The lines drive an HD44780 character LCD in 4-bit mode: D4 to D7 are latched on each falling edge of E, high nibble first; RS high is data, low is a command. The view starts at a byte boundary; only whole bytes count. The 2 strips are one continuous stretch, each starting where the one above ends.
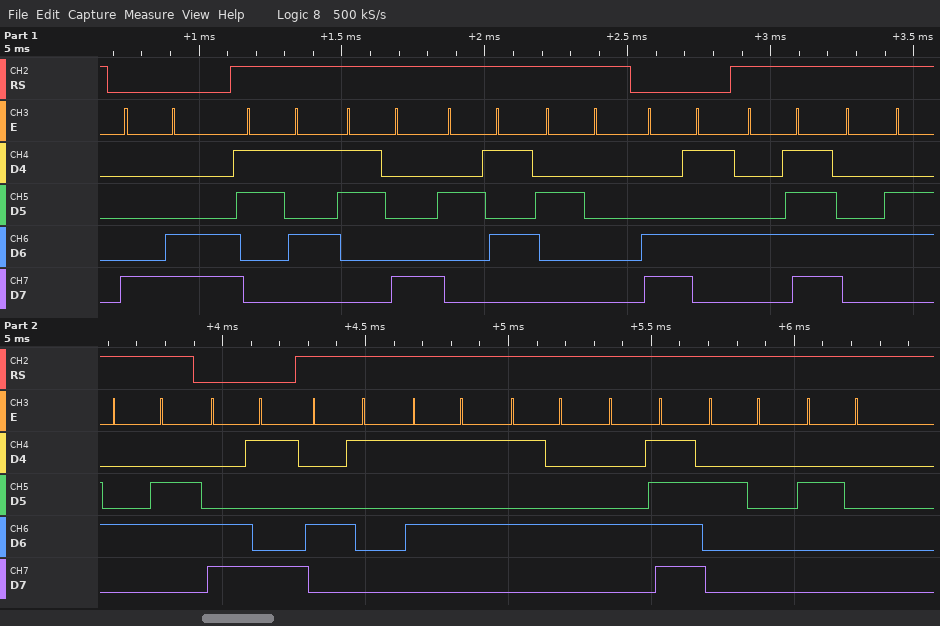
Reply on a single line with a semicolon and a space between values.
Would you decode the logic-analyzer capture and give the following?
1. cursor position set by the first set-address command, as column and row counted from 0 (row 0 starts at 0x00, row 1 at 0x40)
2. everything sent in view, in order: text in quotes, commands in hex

column 12, row 0; 0x8C "58% " 0xC5 "OFF" 0xC9 "AUTO  "
